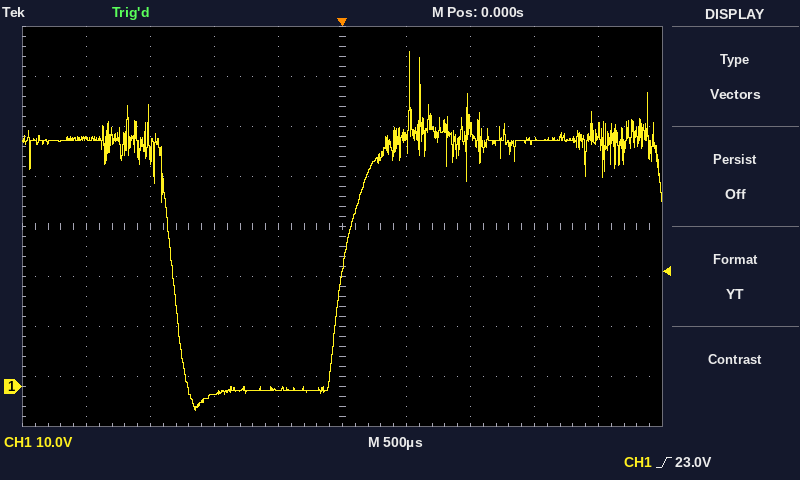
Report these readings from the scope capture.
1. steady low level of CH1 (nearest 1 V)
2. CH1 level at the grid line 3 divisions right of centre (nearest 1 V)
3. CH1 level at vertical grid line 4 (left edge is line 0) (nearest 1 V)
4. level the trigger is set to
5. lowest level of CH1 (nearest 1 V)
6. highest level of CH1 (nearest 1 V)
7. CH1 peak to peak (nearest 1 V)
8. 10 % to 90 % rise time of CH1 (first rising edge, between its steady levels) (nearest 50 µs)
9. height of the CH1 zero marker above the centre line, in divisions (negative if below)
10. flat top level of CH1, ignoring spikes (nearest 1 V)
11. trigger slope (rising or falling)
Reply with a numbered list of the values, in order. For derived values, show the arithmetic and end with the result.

1. -1 V
2. 49 V
3. -1 V
4. 23.0 V
5. -5 V
6. 67 V
7. 67 V − (-5 V) = 72 V
8. 300 µs
9. -3.2 div
10. 49 V
11. rising
